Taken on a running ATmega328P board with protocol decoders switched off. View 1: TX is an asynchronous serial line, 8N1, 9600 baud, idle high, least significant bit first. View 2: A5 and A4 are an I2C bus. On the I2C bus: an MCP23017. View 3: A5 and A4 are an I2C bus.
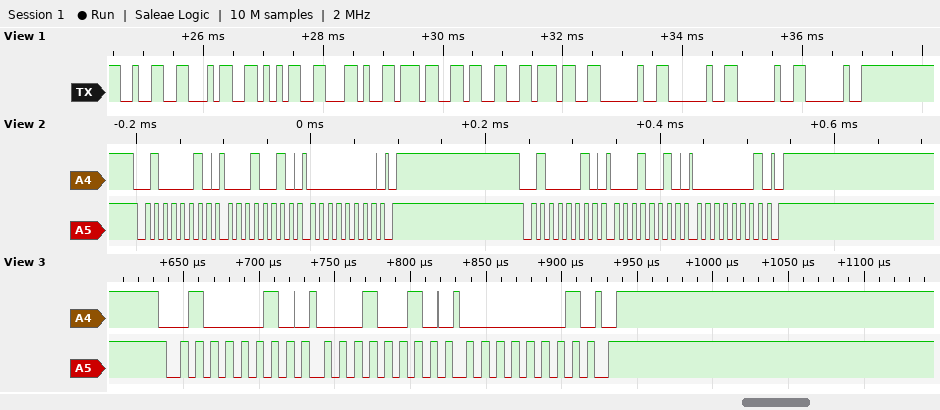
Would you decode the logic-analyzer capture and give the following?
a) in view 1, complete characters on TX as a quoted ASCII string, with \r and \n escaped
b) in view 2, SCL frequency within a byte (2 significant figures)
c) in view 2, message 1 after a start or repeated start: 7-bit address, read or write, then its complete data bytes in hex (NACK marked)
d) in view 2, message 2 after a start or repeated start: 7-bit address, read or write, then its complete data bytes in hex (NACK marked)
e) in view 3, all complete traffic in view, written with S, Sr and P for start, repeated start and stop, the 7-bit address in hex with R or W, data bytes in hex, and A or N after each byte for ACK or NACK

"245,737    "
100 kHz
0x21 write: 12 00
0x21 write: 12 01
S 21W A 12 A 01 A P
